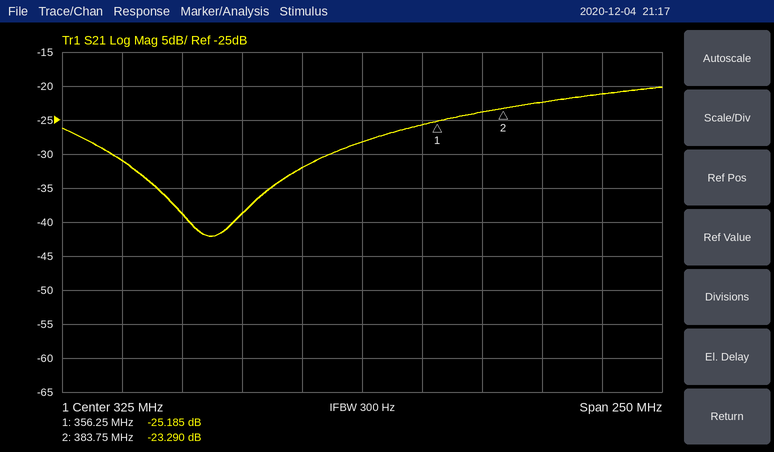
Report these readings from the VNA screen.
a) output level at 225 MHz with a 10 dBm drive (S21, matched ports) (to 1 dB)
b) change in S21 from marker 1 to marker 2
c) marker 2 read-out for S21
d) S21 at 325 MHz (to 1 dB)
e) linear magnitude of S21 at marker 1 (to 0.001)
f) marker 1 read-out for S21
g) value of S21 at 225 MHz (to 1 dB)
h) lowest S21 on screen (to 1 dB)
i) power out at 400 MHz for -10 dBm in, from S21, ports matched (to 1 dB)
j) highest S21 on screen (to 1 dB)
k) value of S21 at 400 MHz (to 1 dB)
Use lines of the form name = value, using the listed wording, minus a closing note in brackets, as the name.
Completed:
output level at 225 MHz with a 10 dBm drive (S21, matched ports) = -21 dBm
change in S21 from marker 1 to marker 2 = 1.895 dB
marker 2 read-out for S21 = -23.290 dB
S21 at 325 MHz = -28 dB
linear magnitude of S21 at marker 1 = 0.055
marker 1 read-out for S21 = -25.185 dB
value of S21 at 225 MHz = -31 dB
lowest S21 on screen = -42 dB
power out at 400 MHz for -10 dBm in, from S21, ports matched = -32 dBm
highest S21 on screen = -20 dB
value of S21 at 400 MHz = -22 dB
